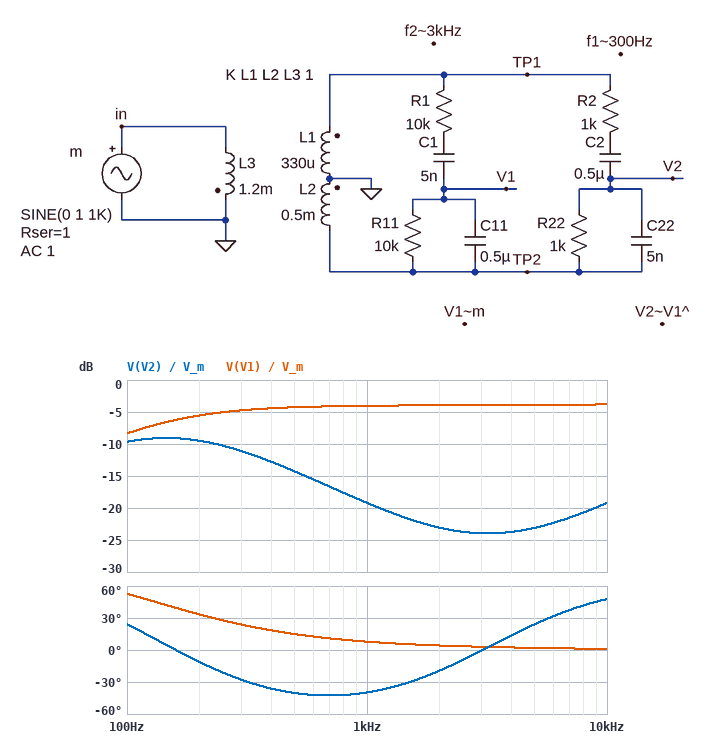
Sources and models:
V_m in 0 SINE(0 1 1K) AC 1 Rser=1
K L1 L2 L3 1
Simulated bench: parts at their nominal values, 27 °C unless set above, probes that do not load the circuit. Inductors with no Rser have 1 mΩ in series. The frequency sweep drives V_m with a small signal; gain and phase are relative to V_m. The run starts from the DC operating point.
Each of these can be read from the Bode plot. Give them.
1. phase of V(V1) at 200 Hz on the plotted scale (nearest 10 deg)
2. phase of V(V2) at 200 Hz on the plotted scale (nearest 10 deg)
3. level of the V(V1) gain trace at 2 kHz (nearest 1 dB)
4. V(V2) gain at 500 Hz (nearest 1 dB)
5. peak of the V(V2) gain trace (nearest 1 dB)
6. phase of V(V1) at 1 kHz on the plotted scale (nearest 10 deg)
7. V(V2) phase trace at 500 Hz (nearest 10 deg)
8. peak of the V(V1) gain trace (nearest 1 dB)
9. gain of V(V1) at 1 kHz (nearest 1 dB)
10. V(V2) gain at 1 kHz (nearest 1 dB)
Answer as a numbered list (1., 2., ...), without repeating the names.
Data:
1. 30 deg
2. -10 deg
3. -4 dB
4. -14 dB
5. -9 dB
6. 10 deg
7. -40 deg
8. -4 dB
9. -4 dB
10. -19 dB
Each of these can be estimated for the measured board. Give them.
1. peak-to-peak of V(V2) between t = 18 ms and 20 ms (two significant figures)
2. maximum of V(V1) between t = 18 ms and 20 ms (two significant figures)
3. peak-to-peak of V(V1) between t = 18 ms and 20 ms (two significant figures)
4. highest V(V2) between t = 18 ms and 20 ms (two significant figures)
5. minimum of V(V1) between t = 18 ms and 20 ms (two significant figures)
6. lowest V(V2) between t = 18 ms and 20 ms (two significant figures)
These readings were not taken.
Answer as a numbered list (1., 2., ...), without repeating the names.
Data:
1. 220 mV
2. 630 mV
3. 1.3 V
4. 110 mV
5. -630 mV
6. -110 mV
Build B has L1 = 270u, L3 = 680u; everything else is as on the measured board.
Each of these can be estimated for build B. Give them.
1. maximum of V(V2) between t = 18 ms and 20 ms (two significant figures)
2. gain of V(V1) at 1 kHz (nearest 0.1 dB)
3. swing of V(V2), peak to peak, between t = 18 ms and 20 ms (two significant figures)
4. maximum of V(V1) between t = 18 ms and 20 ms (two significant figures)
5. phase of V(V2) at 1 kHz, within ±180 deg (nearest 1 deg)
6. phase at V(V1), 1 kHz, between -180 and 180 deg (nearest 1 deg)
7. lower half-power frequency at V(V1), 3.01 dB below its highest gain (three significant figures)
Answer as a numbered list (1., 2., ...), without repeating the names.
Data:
1. 160 mV
2. -1.7 dB
3. 330 mV
4. 820 mV
5. -25 deg
6. 13 deg
7. 242 Hz
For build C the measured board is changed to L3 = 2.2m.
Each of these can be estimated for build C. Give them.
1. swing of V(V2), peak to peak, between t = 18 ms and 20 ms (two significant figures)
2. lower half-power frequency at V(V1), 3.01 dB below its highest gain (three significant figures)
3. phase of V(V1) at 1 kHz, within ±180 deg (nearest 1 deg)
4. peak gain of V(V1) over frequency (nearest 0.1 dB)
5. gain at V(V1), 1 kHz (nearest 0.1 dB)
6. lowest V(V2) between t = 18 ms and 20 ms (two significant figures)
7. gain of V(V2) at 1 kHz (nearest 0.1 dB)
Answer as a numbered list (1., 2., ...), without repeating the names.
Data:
1. 160 mV
2. 74.6 Hz
3. 4 deg
4. -6.4 dB
5. -6.6 dB
6. -82 mV
7. -21.8 dB
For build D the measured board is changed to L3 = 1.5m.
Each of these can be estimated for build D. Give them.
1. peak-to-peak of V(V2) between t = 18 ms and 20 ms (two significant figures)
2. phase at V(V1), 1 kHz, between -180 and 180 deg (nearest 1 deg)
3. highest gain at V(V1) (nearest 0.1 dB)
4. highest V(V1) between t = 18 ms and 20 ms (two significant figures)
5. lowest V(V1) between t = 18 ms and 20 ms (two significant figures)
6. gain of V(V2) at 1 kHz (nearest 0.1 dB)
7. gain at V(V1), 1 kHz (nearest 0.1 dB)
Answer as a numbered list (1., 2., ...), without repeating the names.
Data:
1. 200 mV
2. 6 deg
3. -4.8 dB
4. 560 mV
5. -560 mV
6. -20.1 dB
7. -5.0 dB
